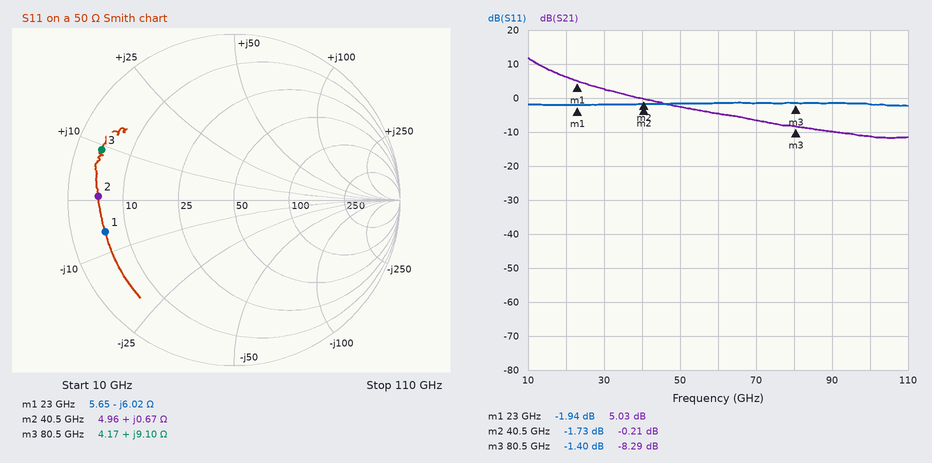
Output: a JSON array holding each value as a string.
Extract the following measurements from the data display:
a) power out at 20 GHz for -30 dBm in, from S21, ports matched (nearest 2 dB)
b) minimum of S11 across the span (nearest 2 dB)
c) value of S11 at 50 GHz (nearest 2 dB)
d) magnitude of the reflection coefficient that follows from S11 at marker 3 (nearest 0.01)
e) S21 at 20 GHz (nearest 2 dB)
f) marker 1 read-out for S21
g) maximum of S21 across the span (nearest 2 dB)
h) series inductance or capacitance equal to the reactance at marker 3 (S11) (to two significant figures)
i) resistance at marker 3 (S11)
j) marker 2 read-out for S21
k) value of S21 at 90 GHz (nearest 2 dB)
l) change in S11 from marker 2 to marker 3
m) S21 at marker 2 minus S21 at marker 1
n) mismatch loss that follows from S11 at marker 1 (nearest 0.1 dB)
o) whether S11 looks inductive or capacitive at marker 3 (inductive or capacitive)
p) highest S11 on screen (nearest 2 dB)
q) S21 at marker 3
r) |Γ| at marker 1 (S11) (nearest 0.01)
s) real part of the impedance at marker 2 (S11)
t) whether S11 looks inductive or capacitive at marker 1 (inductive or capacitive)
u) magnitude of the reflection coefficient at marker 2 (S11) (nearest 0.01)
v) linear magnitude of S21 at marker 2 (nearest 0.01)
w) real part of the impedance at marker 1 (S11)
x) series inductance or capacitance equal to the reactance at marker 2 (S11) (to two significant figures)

["-24 dBm", "-2 dB", "-2 dB", "0.85", "6 dB", "5.03 dB", "12 dB", "18 pH", "4.17 Ω", "-0.21 dB", "-10 dB", "0.33 dB", "-5.24 dB", "4.4 dB", "inductive", "-2 dB", "-8.29 dB", "0.80", "4.96 Ω", "capacitive", "0.82", "0.98", "5.65 Ω", "2.6 pH"]
